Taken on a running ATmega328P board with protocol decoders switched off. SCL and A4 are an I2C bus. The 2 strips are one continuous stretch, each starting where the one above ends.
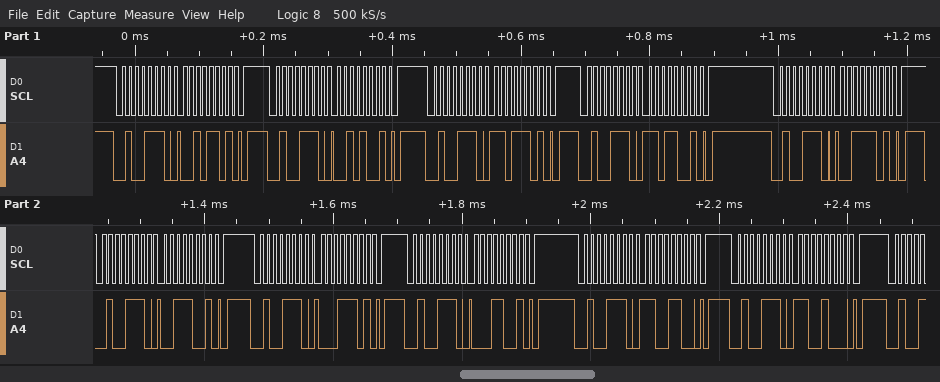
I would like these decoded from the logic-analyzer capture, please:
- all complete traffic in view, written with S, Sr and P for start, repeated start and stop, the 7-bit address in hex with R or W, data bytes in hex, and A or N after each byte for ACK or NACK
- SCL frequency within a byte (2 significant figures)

S 27W A 2D A P S 27W A 29 A P S 27W A DD A P S 27W A D9 A P S 27W A 3D A P S 27W A 39 A P S 27W A 1D A P S 27W A 19 A P S 27W A CC A P S 27W A C8 A P
100 kHz
